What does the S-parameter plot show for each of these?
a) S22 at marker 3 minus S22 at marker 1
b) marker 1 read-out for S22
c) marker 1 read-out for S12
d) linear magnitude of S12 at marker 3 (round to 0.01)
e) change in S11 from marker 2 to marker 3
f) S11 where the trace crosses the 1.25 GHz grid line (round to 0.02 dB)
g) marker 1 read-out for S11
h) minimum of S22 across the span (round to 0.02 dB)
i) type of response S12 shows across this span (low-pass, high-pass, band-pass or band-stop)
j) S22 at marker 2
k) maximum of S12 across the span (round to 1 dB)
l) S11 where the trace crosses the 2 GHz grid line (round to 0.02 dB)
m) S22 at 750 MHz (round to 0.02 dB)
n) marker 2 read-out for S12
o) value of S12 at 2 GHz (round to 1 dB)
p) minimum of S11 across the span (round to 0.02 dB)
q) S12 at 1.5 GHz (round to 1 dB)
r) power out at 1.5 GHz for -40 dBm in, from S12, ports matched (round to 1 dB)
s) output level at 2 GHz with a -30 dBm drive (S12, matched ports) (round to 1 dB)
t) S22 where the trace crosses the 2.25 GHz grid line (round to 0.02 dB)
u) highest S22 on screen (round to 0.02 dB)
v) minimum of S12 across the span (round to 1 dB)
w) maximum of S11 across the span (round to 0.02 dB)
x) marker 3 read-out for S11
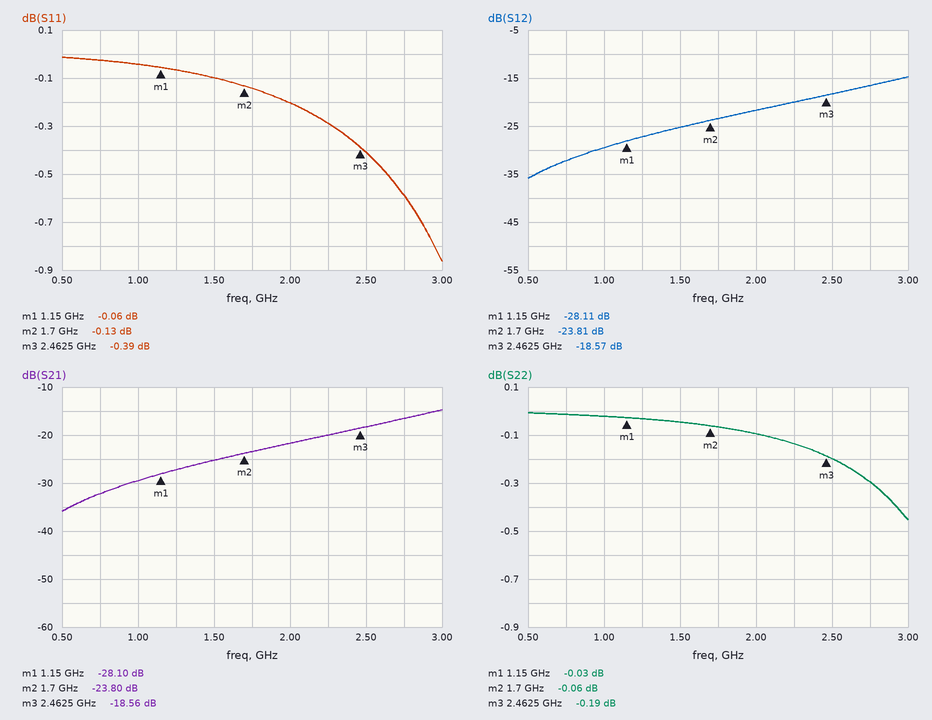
-0.16 dB
-0.03 dB
-28.11 dB
0.12
-0.26 dB
-0.06 dB
-0.06 dB
-0.46 dB
high-pass
-0.06 dB
-15 dB
-0.20 dB
-0.02 dB
-23.81 dB
-22 dB
-0.86 dB
-25 dB
-65 dBm
-52 dBm
-0.14 dB
0.00 dB
-36 dB
-0.02 dB
-0.39 dB
